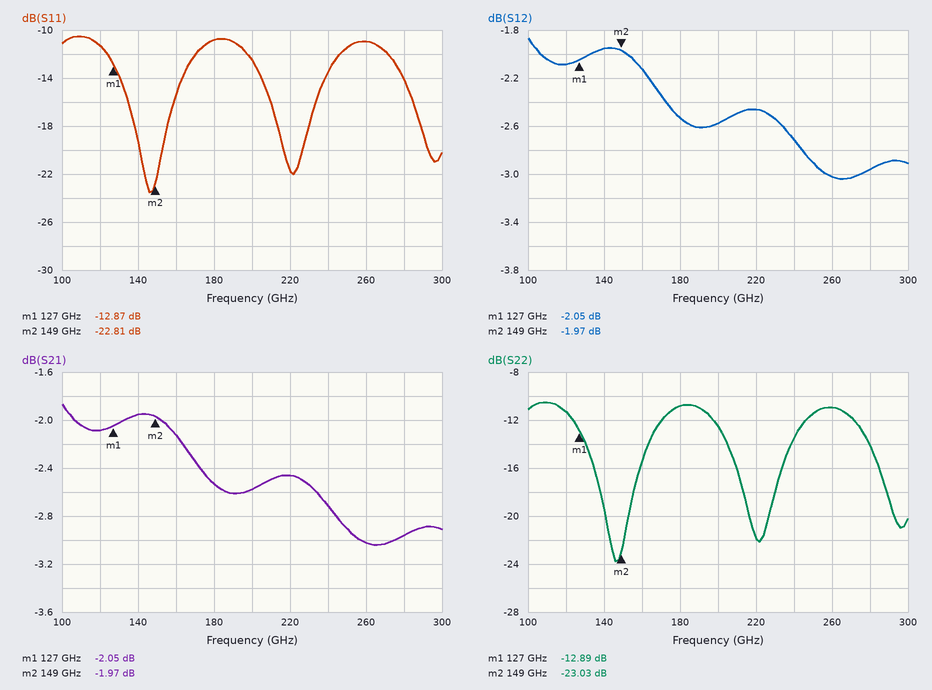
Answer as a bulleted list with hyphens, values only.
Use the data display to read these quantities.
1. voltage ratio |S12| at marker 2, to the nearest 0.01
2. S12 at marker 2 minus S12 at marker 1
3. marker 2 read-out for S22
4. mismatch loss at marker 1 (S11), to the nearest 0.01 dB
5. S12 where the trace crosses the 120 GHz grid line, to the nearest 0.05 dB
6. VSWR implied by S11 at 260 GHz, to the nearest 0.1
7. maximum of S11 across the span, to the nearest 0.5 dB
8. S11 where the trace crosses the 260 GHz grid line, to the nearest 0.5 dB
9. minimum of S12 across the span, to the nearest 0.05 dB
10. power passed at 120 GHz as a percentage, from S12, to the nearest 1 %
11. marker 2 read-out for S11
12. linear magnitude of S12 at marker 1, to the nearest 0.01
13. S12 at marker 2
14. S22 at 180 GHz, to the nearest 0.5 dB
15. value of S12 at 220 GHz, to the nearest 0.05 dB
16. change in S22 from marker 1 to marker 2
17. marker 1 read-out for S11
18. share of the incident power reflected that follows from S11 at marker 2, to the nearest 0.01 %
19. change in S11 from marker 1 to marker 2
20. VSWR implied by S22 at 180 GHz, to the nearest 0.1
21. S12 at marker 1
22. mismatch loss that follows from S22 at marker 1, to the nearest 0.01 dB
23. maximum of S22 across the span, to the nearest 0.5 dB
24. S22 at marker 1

- 0.80
- 0.08 dB
- -23.03 dB
- 0.23 dB
- -2.10 dB
- 1.8
- -10.5 dB
- -11.0 dB
- -3.05 dB
- 62 %
- -22.81 dB
- 0.79
- -1.97 dB
- -11.0 dB
- -2.45 dB
- -10.14 dB
- -12.87 dB
- 0.52 %
- -9.94 dB
- 1.8
- -2.05 dB
- 0.23 dB
- -10.5 dB
- -12.89 dB
